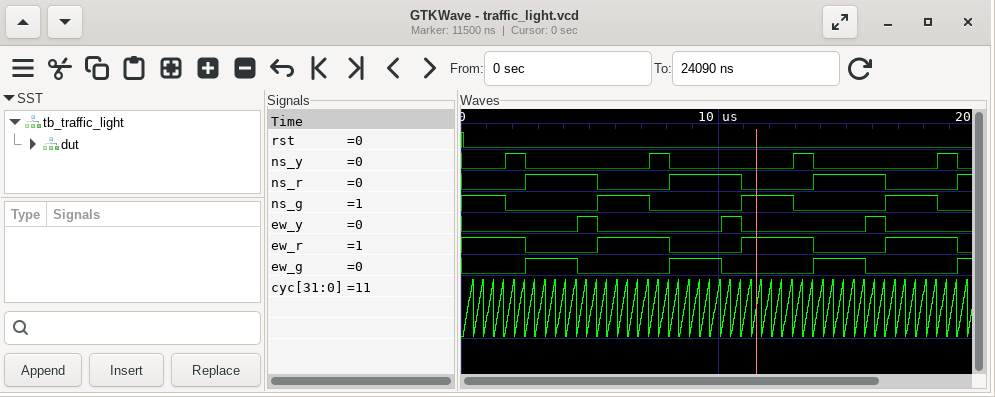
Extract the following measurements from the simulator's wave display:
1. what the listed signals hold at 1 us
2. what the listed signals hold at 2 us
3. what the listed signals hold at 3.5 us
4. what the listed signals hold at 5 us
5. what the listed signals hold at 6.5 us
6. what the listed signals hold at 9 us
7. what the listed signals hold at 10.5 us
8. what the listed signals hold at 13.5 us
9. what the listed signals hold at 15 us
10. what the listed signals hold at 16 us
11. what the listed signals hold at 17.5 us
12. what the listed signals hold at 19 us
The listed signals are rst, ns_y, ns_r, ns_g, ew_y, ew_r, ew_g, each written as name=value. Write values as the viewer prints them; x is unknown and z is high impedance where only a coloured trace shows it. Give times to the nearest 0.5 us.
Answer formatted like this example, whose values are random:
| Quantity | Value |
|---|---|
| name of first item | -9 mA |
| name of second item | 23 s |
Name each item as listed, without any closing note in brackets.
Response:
| Quantity | Value |
|---|---|
| what the listed signals hold at 1 us | rst=0, ns_y=0, ns_r=0, ns_g=1, ew_y=0, ew_r=1, ew_g=0 |
| what the listed signals hold at 2 us | rst=0, ns_y=1, ns_r=0, ns_g=0, ew_y=0, ew_r=1, ew_g=0 |
| what the listed signals hold at 3.5 us | rst=0, ns_y=0, ns_r=1, ns_g=0, ew_y=0, ew_r=0, ew_g=1 |
| what the listed signals hold at 5 us | rst=0, ns_y=0, ns_r=1, ns_g=0, ew_y=1, ew_r=0, ew_g=0 |
| what the listed signals hold at 6.5 us | rst=0, ns_y=0, ns_r=0, ns_g=1, ew_y=0, ew_r=1, ew_g=0 |
| what the listed signals hold at 9 us | rst=0, ns_y=0, ns_r=1, ns_g=0, ew_y=0, ew_r=0, ew_g=1 |
| what the listed signals hold at 10.5 us | rst=0, ns_y=0, ns_r=1, ns_g=0, ew_y=1, ew_r=0, ew_g=0 |
| what the listed signals hold at 13.5 us | rst=0, ns_y=1, ns_r=0, ns_g=0, ew_y=0, ew_r=1, ew_g=0 |
| what the listed signals hold at 15 us | rst=0, ns_y=0, ns_r=1, ns_g=0, ew_y=0, ew_r=0, ew_g=1 |
| what the listed signals hold at 16 us | rst=0, ns_y=0, ns_r=1, ns_g=0, ew_y=1, ew_r=0, ew_g=0 |
| what the listed signals hold at 17.5 us | rst=0, ns_y=0, ns_r=0, ns_g=1, ew_y=0, ew_r=1, ew_g=0 |
| what the listed signals hold at 19 us | rst=0, ns_y=1, ns_r=0, ns_g=0, ew_y=0, ew_r=1, ew_g=0 |
